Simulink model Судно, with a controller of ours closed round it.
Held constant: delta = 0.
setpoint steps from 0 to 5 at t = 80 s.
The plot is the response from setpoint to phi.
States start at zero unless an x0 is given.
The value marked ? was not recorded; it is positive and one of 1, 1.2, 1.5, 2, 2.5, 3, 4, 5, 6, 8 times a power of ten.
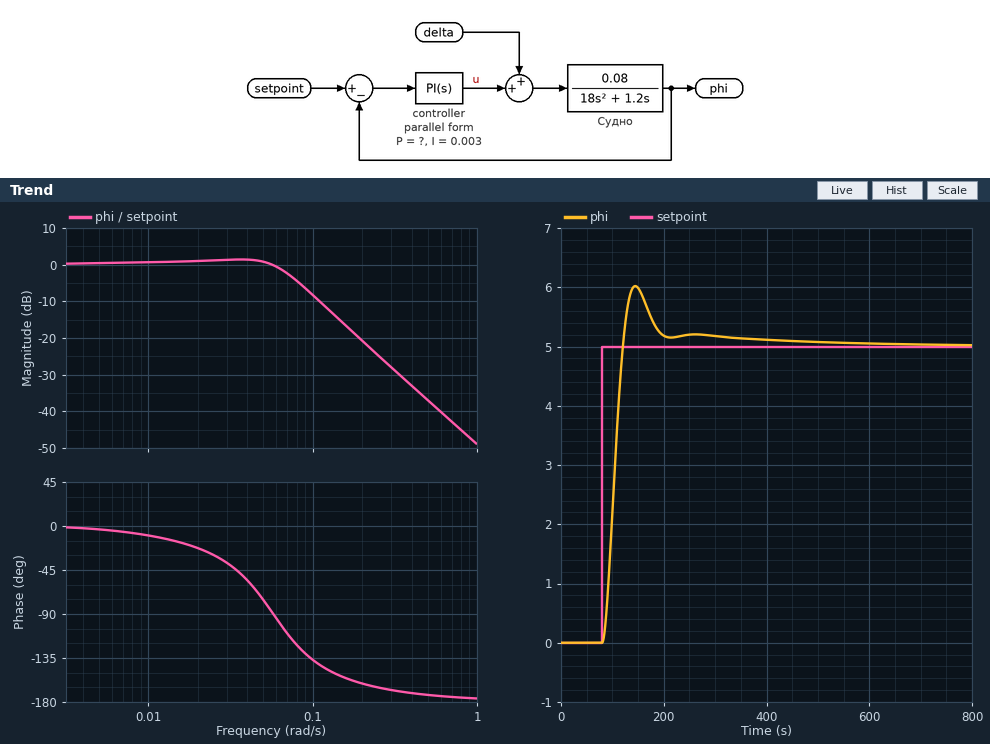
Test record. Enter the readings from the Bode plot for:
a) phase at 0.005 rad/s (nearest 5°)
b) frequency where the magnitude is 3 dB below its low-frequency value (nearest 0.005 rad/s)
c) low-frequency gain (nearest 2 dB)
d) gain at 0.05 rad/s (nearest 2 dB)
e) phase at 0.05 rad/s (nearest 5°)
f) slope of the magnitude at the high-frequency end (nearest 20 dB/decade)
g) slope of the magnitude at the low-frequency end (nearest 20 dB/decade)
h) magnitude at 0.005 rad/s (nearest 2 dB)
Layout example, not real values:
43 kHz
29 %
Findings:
-5°
0.070 rad/s
0 dB
0 dB
-75°
-40 dB/decade
0 dB/decade
0 dB
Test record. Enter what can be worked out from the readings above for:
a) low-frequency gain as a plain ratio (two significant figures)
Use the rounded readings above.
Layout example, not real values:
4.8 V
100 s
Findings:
1.0
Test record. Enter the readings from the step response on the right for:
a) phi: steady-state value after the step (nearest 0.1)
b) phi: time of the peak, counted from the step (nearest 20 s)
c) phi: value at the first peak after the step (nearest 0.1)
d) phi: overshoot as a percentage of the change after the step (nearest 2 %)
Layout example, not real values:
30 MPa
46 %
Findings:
5.0
60 s
6.0
20 %
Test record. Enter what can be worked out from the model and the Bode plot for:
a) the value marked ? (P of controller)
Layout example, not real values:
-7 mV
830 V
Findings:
0.8
